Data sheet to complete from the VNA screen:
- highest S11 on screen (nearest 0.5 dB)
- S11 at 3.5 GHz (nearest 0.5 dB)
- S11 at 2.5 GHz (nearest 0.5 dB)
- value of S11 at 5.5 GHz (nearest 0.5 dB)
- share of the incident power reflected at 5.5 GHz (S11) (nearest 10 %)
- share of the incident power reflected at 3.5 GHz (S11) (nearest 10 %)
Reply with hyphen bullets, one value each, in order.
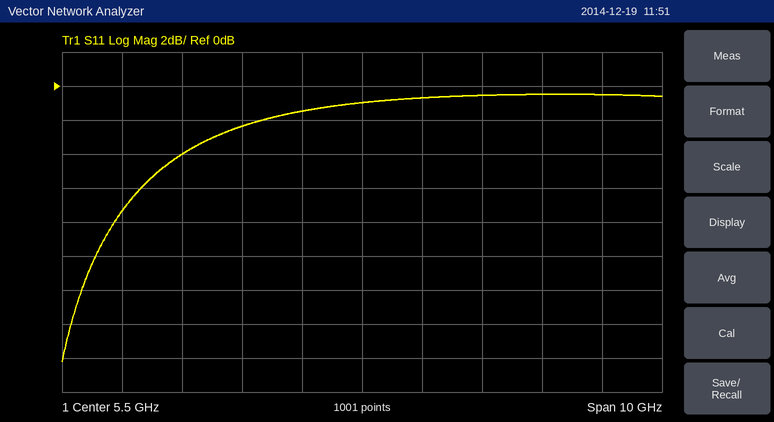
- -0.5 dB
- -2.5 dB
- -4.0 dB
- -1.0 dB
- 80 %
- 60 %
